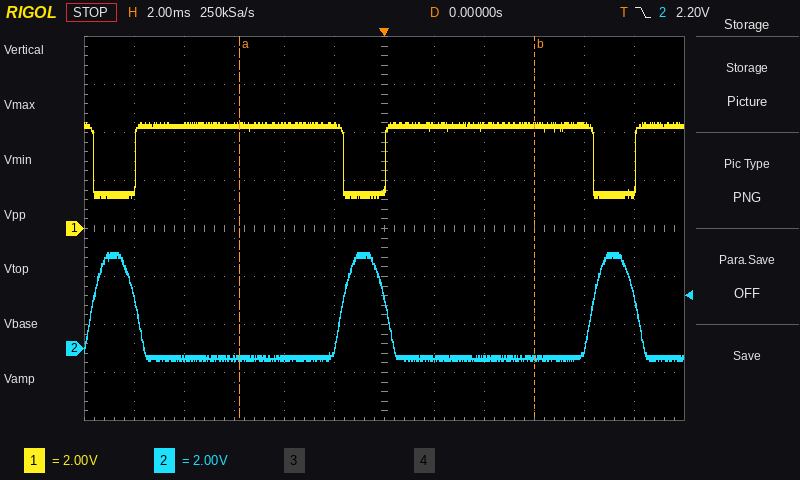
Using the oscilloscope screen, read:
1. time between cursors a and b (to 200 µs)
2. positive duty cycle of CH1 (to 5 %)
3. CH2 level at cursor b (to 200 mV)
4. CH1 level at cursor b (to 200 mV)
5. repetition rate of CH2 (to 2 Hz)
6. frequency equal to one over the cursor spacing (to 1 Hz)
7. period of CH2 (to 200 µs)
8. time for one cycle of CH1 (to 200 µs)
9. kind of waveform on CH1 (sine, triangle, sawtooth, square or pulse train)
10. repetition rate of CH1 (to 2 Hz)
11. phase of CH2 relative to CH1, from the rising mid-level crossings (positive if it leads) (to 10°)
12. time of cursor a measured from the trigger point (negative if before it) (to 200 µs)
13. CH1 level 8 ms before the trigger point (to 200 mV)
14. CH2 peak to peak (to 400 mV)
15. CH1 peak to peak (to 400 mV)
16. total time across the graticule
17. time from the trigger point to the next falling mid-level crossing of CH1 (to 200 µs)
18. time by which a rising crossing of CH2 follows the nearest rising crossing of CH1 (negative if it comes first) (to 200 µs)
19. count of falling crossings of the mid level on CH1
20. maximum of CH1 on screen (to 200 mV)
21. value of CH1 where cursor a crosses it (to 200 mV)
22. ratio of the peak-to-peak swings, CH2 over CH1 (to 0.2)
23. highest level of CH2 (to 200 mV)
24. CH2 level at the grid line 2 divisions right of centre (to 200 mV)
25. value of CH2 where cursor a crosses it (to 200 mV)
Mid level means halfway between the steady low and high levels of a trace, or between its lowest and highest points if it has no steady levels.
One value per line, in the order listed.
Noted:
11.8 ms
85 %
-400 mV
4.4 V
100 Hz
85 Hz
10.0 ms
10.0 ms
pulse train
100 Hz
+60°
-5.8 ms
4.4 V
4.4 V
3.2 V
24 ms
8.4 ms
-1.8 ms
3
4.4 V
4.4 V
1.4
4.0 V
-400 mV
-400 mV
